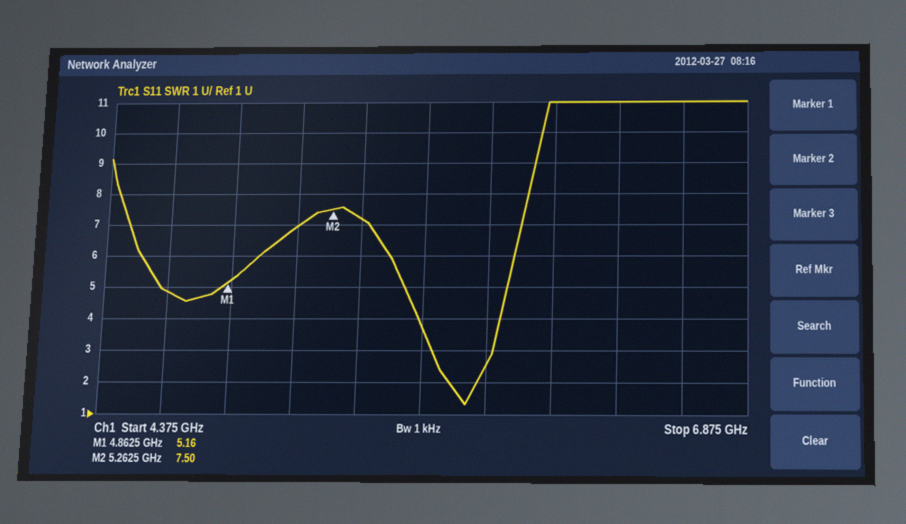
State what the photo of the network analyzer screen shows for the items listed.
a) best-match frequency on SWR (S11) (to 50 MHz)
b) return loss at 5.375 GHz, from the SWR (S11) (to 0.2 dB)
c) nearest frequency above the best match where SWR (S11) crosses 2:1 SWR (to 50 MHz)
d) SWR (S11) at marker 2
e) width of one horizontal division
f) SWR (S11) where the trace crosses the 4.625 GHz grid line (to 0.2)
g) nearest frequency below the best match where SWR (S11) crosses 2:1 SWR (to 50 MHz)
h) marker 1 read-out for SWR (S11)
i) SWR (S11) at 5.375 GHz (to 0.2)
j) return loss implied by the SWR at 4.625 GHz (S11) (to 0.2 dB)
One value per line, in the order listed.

5.80 GHz
2.4 dB
5.85 GHz
7.50
250 MHz
4.8
5.75 GHz
5.16
7.2
3.6 dB
